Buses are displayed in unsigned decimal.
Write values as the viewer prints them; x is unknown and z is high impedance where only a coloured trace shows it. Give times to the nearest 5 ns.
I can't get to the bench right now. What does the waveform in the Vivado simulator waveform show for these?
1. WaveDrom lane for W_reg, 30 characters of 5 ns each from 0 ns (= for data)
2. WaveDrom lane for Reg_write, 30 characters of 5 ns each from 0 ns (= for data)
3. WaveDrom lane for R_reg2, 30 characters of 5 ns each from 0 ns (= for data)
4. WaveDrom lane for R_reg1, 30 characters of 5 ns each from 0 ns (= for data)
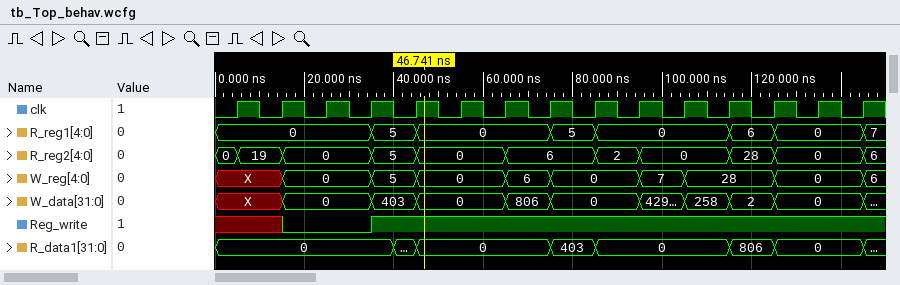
{name: 'W_reg', wave: 'x..=...=.=...=.=...=.=...=...=', data: '0 5 0 6 0 7 28 0 6'}
{name: 'Reg_write', wave: 'x..0...1......................'}
{name: 'R_reg2', wave: '==.=...=.=...=...=.=...=.=...=', data: '0 19 0 5 0 6 2 0 28 0 6'}
{name: 'R_reg1', wave: '=......=.=.....=.=.....=.=...=', data: '0 5 0 5 0 6 0 7'}
